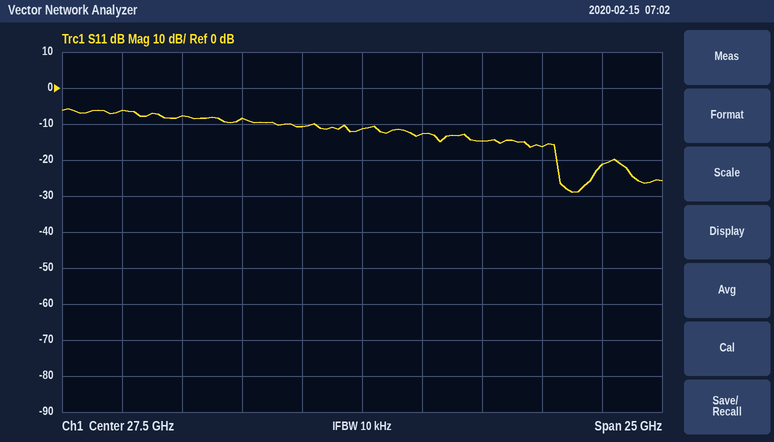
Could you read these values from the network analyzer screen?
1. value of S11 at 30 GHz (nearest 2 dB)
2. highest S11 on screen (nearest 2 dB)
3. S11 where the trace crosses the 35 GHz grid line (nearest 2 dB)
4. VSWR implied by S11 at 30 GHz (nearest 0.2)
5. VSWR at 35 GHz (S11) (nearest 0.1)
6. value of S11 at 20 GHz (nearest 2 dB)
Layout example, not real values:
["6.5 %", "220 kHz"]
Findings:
["-12 dB", "-6 dB", "-16 dB", "1.6", "1.4", "-8 dB"]
